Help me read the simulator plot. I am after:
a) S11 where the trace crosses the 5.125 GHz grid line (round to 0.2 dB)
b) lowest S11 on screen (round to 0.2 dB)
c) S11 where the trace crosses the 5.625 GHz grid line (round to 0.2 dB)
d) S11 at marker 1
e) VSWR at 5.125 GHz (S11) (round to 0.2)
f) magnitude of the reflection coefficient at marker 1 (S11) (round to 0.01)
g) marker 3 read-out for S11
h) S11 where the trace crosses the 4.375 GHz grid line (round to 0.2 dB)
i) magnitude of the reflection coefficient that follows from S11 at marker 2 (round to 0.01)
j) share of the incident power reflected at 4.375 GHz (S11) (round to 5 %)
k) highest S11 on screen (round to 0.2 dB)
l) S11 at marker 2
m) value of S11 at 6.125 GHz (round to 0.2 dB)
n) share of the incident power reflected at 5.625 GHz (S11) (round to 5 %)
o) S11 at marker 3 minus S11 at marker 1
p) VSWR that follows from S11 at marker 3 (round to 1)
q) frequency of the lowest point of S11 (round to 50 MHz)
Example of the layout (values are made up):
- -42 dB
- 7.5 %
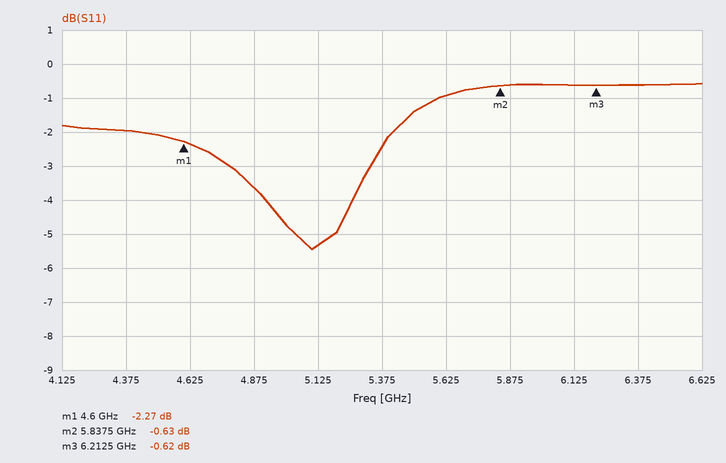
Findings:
- -5.4 dB
- -5.4 dB
- -1.0 dB
- -2.27 dB
- 3.4
- 0.77
- -0.62 dB
- -2.0 dB
- 0.93
- 65 %
- -0.6 dB
- -0.63 dB
- -0.6 dB
- 80 %
- 1.65 dB
- 28
- 5.10 GHz
